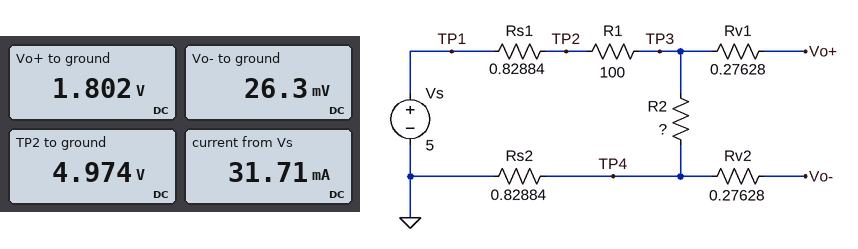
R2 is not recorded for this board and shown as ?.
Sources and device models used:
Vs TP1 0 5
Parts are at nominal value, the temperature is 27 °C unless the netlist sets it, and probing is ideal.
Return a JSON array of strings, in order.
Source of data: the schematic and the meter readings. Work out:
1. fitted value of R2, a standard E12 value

["56 Ω"]
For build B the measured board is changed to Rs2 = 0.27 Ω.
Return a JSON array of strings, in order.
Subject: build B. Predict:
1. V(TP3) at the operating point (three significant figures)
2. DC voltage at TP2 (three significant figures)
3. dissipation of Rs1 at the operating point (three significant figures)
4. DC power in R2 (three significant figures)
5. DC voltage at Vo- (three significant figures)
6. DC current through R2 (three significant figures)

["1.79 V", "4.97 V", "840 µW", "56.7 mW", "8.59 mV", "31.8 mA"]
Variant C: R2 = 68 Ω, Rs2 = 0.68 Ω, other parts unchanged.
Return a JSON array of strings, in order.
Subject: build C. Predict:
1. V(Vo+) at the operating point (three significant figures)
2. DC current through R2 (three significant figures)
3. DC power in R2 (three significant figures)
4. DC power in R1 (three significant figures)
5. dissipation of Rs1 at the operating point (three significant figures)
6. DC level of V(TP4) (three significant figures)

["2.03 V", "29.5 mA", "59.2 mW", "87.0 mW", "721 µW", "20.1 mV"]
